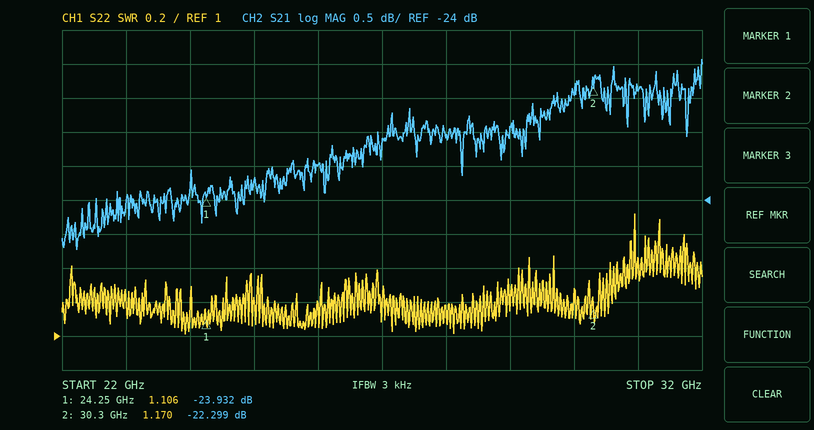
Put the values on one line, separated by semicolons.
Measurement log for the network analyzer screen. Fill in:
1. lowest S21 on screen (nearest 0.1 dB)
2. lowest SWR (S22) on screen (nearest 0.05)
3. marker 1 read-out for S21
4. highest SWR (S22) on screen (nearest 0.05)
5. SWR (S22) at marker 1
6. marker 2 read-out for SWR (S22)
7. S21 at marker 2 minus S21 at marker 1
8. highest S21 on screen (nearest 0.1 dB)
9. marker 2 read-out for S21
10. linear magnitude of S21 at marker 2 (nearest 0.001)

-24.7 dB; 1.00; -23.932 dB; 1.70; 1.106; 1.170; 1.633 dB; -21.9 dB; -22.299 dB; 0.077
